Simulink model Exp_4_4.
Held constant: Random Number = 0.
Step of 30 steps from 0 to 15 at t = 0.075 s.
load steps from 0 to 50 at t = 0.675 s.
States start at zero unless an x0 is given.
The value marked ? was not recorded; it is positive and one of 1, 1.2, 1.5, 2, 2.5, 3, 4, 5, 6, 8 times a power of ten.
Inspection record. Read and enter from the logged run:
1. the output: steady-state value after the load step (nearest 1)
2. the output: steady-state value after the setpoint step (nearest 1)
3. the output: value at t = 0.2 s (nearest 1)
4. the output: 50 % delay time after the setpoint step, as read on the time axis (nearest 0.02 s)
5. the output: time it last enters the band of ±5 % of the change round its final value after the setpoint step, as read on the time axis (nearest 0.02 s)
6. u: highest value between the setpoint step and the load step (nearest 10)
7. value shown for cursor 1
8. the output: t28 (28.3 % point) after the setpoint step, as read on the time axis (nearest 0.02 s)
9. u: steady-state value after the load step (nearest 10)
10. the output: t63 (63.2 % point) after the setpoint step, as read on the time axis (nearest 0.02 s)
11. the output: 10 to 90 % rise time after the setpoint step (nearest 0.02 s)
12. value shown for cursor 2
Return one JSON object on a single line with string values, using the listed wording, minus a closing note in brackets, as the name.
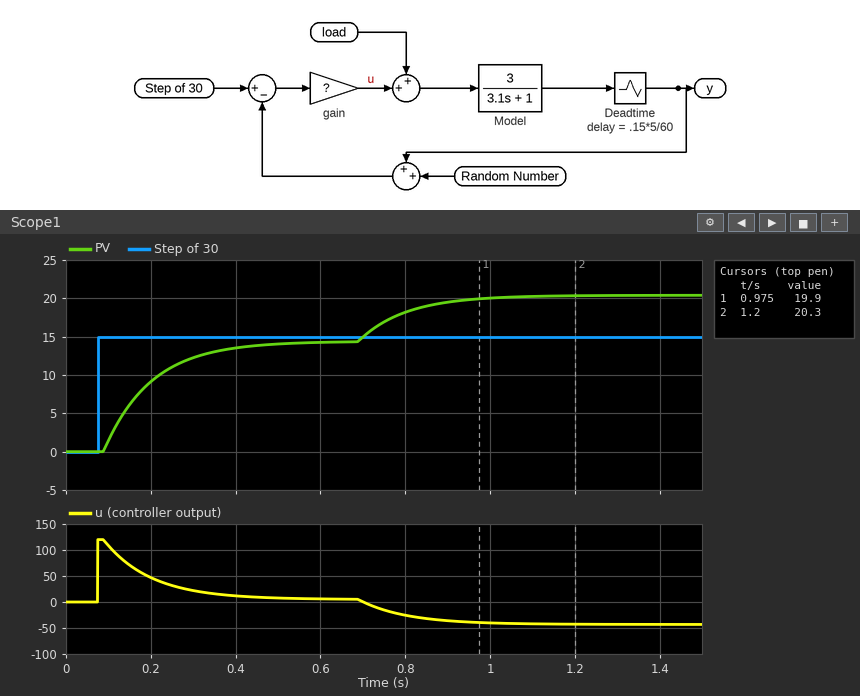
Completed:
{"the output: steady-state value after the load step": "20", "the output: steady-state value after the setpoint step": "14", "the output: value at t = 0.2 s": "9", "the output: 50 % delay time after the setpoint step, as read on the time axis": "0.16 s", "the output: time it last enters the band of ±5 % of the change round its final value after the setpoint step, as read on the time axis": "0.42 s", "u: highest value between the setpoint step and the load step": "120", "value shown for cursor 1": "19.9", "the output: t28 (28.3 % point) after the setpoint step, as read on the time axis": "0.12 s", "u: steady-state value after the load step": "-40", "the output: t63 (63.2 % point) after the setpoint step, as read on the time axis": "0.20 s", "the output: 10 to 90 % rise time after the setpoint step": "0.24 s", "value shown for cursor 2": "20.3"}
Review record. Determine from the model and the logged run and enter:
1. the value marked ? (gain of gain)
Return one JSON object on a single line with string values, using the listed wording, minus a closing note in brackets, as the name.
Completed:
{"the value marked ?": "8"}
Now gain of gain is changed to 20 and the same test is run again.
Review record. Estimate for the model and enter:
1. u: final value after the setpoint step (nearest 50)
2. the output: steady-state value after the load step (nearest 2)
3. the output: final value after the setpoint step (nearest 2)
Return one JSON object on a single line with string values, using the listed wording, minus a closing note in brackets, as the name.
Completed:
{"u: final value after the setpoint step": "0", "the output: steady-state value after the load step": "18", "the output: final value after the setpoint step": "14"}
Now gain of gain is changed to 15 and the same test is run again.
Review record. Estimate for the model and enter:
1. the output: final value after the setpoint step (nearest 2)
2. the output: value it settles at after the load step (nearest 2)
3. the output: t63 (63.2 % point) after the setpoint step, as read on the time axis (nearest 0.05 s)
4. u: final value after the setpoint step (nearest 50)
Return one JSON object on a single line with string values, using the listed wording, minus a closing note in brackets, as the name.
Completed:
{"the output: final value after the setpoint step": "14", "the output: value it settles at after the load step": "18", "the output: t63 (63.2 % point) after the setpoint step, as read on the time axis": "0.15 s", "u: final value after the setpoint step": "0"}
